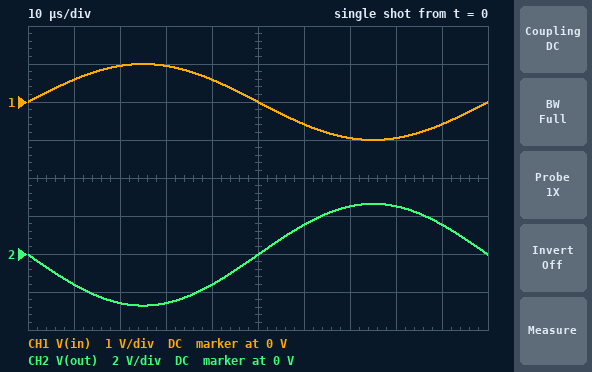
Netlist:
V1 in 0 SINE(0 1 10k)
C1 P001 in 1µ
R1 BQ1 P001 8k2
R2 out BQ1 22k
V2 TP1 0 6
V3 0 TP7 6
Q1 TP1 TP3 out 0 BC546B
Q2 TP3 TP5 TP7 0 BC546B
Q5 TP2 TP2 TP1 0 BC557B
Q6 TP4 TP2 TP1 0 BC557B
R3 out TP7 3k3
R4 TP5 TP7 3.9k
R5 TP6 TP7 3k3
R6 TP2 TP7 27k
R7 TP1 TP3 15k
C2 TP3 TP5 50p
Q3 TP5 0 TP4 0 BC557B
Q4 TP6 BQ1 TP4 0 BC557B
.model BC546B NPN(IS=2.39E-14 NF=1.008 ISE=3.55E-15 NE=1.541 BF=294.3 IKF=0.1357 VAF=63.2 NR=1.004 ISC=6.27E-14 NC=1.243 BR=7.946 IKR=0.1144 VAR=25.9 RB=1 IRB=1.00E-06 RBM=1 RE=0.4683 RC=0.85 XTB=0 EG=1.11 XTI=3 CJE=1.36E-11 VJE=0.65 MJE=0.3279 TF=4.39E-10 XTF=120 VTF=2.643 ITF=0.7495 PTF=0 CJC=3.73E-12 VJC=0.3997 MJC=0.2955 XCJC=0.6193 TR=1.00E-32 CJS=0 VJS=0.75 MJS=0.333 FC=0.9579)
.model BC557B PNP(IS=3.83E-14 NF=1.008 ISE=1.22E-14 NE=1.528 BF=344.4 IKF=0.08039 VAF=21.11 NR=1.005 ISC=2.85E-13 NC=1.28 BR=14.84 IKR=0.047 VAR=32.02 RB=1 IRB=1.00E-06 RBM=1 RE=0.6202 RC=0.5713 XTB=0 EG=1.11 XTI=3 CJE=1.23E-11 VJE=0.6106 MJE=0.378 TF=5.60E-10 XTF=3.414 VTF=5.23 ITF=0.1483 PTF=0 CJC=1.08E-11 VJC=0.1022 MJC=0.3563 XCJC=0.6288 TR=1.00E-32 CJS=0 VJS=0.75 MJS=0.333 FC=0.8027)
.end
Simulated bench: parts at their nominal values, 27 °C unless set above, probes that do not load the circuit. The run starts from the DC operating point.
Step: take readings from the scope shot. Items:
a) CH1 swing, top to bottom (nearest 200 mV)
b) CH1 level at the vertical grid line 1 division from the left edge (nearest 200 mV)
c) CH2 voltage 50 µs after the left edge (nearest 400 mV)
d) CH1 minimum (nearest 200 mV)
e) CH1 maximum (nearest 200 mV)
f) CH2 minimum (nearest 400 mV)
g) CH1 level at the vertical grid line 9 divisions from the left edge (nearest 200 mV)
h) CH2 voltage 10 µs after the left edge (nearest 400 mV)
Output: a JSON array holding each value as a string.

["2.0 V", "600 mV", "0 V", "-1.0 V", "1.0 V", "-2.8 V", "-600 mV", "-1.6 V"]
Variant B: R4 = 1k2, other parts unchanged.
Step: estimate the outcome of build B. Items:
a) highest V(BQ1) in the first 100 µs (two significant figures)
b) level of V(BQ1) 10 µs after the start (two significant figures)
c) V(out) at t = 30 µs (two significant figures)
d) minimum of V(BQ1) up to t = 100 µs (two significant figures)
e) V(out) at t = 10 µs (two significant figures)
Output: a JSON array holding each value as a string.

["510 mV", "340 mV", "-1.2 V", "78 mV", "-640 mV"]
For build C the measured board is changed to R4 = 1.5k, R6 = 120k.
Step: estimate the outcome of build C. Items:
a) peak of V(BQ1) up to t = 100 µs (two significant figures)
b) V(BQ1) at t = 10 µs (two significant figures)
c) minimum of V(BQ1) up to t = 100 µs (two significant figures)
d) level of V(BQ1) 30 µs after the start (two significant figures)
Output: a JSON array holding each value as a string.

["5.9 V", "5.6 V", "4.4 V", "5.8 V"]
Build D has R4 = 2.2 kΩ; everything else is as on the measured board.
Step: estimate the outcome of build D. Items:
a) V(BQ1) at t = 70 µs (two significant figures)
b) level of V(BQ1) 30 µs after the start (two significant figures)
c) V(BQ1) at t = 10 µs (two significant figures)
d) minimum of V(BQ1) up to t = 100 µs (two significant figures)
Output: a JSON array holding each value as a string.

["1.5 mV", "4.7 mV", "6.4 mV", "1.3 mV"]
